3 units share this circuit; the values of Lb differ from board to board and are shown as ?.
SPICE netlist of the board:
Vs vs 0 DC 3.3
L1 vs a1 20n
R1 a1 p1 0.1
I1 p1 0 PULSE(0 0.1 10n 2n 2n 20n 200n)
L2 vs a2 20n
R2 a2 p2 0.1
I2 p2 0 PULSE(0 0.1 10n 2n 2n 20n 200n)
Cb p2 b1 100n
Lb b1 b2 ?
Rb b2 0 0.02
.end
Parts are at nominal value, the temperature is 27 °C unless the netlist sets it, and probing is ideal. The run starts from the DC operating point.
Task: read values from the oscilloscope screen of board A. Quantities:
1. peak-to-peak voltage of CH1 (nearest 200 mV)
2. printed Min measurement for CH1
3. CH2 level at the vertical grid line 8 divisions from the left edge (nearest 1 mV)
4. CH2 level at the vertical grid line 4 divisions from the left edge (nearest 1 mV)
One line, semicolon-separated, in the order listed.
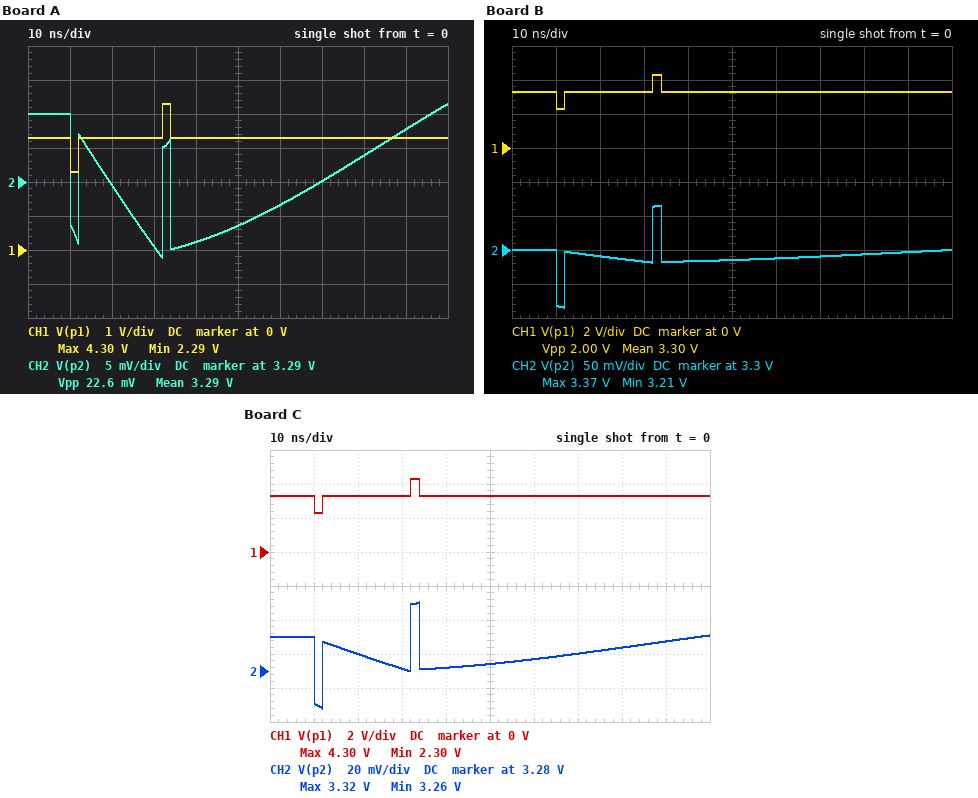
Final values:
2.0 V; 2.29 V; 3.294 V; 3.281 V
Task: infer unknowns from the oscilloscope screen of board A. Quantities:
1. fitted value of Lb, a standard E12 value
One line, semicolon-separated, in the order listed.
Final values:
330 pH
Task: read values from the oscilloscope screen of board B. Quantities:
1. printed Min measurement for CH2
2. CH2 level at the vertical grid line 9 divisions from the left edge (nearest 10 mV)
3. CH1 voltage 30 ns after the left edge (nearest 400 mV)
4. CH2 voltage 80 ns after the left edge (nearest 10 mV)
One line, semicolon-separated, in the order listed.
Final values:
3.21 V; 3.30 V; 3.2 V; 3.29 V
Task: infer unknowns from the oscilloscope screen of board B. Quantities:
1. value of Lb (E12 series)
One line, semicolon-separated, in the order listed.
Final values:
1.8 nH
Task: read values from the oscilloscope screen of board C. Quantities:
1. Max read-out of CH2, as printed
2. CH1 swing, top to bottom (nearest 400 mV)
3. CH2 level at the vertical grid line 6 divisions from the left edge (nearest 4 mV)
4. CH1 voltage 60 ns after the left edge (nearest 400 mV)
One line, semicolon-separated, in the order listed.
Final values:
3.32 V; 2.0 V; 3.288 V; 3.2 V
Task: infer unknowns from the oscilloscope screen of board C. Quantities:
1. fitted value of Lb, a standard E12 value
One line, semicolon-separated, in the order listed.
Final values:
820 pH
